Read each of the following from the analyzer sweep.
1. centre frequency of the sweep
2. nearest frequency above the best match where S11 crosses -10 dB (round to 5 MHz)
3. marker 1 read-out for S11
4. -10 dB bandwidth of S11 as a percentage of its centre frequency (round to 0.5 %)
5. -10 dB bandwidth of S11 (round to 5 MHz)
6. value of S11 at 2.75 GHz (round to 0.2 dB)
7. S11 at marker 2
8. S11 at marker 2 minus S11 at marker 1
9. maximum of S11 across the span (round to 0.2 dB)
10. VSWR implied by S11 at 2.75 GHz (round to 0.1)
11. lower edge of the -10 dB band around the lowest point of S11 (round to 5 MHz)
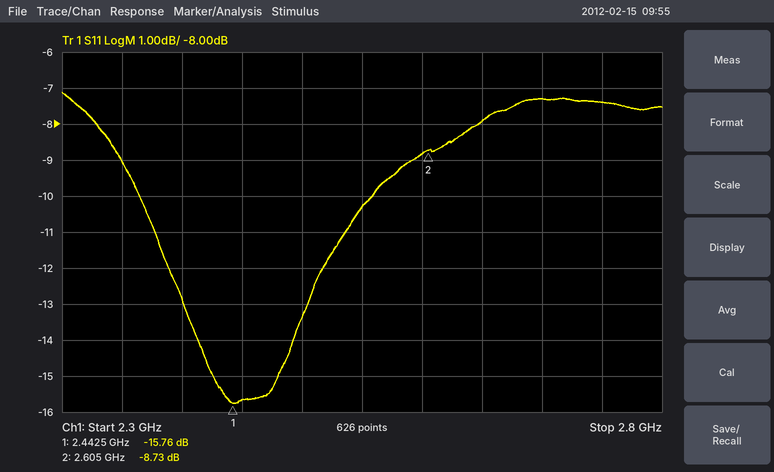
2.55 GHz
2.560 GHz
-15.76 dB
8.0 %
195 MHz
-7.4 dB
-8.73 dB
7.03 dB
-7.2 dB
2.5
2.365 GHz
